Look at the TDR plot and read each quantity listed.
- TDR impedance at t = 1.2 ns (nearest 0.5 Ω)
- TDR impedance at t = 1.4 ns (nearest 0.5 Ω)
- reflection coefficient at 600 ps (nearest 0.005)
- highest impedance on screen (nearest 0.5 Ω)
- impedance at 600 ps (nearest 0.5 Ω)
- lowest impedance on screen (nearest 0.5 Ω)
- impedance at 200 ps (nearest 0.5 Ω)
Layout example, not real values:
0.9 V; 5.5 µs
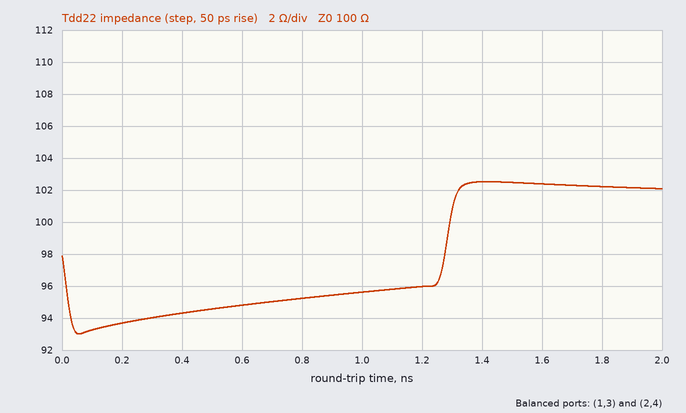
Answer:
96.0 Ω; 102.5 Ω; -0.025; 102.5 Ω; 95.0 Ω; 93.0 Ω; 93.5 Ω
